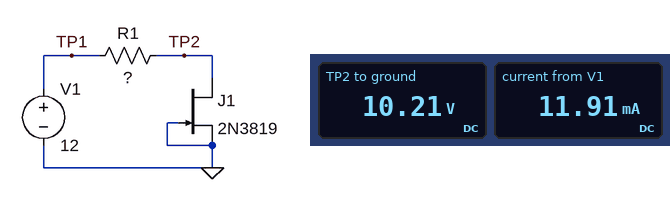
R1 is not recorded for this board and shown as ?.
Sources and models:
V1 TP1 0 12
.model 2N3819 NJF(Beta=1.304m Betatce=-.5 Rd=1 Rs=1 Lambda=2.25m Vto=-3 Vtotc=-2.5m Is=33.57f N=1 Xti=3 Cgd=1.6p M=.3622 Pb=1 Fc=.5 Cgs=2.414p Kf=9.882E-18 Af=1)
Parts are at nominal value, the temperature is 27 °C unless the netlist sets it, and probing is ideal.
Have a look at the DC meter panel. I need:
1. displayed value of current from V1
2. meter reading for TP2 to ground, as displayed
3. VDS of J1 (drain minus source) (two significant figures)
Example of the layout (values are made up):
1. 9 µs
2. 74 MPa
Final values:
1. 11.91 mA
2. 10.21 V
3. 10 V
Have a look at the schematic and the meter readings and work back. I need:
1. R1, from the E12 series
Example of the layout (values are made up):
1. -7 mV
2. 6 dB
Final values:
1. 150 Ω
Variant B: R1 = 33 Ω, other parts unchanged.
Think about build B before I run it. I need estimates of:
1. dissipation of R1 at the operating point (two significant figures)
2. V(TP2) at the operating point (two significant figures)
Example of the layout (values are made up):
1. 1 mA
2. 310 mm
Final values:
1. 4.7 mW
2. 12 V
